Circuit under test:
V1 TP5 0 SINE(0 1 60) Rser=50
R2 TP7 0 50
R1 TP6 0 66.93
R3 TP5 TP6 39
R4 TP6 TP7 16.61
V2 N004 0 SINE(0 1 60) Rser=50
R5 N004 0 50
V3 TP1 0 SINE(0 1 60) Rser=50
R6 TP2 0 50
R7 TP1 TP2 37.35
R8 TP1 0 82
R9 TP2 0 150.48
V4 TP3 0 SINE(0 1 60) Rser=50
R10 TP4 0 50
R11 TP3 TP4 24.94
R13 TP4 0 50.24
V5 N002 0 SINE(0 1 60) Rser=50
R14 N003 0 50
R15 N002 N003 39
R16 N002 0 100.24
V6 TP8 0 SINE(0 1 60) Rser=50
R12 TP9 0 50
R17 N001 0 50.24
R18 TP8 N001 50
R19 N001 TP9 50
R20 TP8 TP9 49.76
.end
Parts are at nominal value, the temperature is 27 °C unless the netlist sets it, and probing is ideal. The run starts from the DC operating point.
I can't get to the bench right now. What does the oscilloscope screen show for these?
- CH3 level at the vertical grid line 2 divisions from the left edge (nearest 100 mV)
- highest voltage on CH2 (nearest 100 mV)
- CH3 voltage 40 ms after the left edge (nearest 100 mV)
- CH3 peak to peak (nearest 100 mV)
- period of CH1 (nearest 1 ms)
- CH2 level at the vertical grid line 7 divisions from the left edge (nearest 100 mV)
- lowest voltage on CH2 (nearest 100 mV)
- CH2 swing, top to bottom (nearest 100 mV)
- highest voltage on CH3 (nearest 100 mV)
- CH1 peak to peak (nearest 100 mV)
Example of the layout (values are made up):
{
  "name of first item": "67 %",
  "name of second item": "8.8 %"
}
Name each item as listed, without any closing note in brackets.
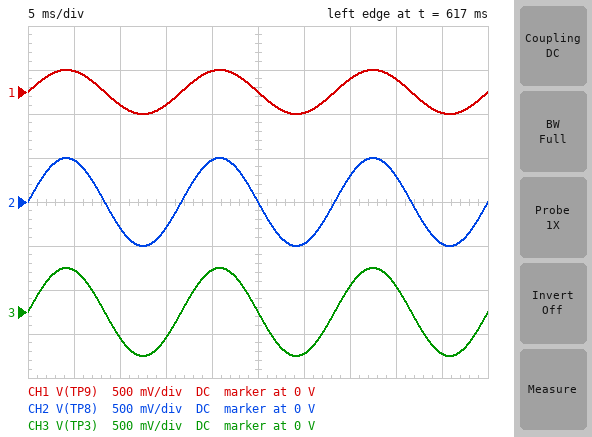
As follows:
{
  "CH3 level at the vertical grid line 2 divisions from the left edge": "-300 mV",
  "highest voltage on CH2": "500 mV",
  "CH3 voltage 40 ms after the left edge": "300 mV",
  "CH3 peak to peak": "1.0 V",
  "period of CH1": "17 ms",
  "CH2 level at the vertical grid line 7 divisions from the left edge": "300 mV",
  "lowest voltage on CH2": "-500 mV",
  "CH2 swing, top to bottom": "1.0 V",
  "highest voltage on CH3": "500 mV",
  "CH1 peak to peak": "500 mV"
}
